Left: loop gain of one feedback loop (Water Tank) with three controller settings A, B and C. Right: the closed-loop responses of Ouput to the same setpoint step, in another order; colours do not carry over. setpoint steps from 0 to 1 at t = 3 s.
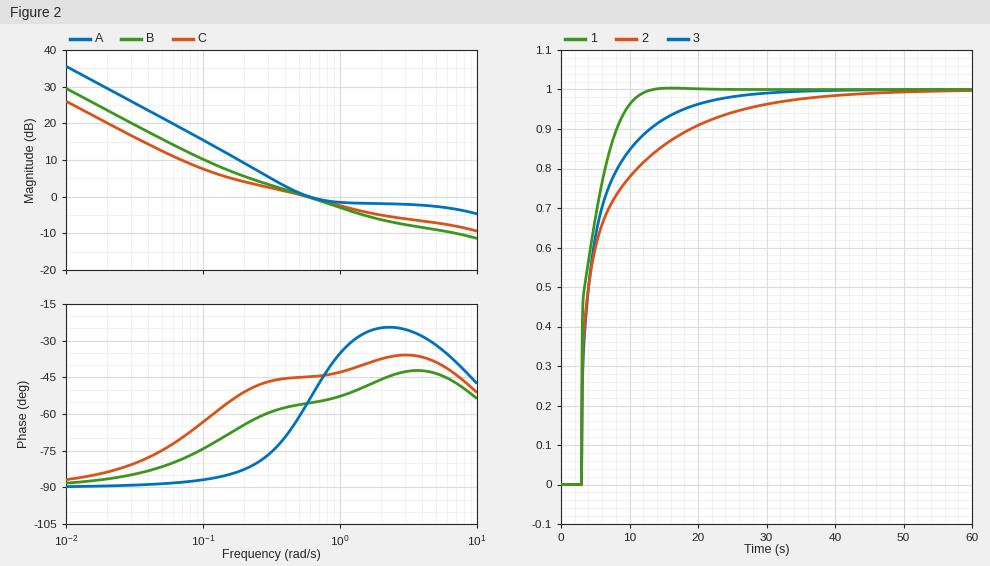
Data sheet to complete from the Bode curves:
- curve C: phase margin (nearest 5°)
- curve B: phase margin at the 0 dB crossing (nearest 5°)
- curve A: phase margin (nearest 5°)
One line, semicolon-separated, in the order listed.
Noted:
135°; 125°; 125°
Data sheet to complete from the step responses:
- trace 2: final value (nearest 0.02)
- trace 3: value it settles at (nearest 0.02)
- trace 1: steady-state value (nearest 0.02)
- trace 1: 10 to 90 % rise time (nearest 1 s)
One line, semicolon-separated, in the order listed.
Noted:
1.00; 1.00; 1.00; 5 s
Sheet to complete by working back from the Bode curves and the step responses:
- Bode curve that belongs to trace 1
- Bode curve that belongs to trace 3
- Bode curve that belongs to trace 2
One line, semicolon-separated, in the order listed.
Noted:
A; B; C
